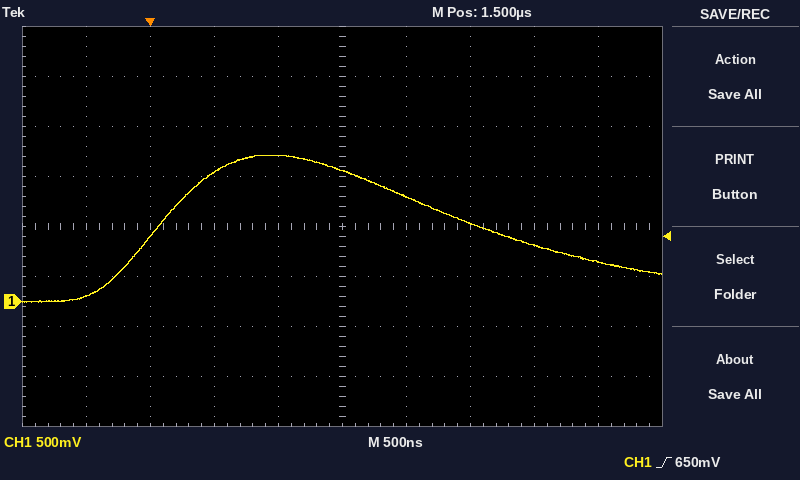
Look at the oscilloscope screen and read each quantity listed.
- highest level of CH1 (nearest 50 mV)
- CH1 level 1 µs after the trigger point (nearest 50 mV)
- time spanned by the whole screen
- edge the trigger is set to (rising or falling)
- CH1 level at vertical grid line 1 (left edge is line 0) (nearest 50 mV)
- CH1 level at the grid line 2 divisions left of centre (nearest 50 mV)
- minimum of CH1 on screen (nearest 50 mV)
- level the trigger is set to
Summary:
1.45 V
1.45 V
5 µs
rising
50 mV
1.30 V
0 mV
650 mV
